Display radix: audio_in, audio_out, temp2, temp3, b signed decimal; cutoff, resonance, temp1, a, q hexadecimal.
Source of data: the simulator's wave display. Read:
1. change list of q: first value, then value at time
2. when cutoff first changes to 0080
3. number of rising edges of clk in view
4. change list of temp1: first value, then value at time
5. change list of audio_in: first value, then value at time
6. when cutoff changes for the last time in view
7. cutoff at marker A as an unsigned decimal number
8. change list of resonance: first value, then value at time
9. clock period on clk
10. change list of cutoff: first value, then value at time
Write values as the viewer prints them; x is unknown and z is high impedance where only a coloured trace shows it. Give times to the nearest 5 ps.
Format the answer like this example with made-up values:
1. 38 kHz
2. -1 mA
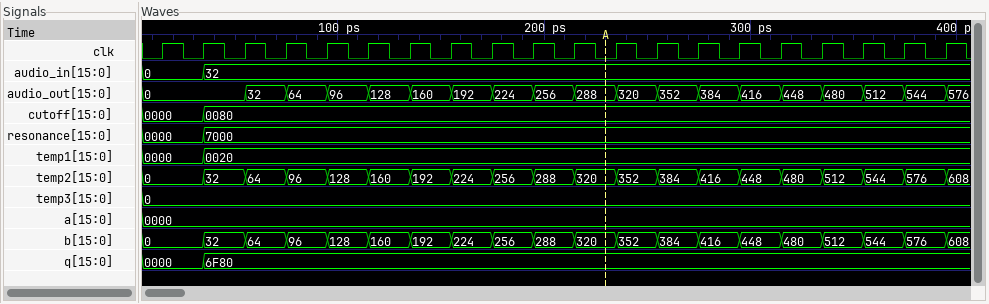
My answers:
1. 0000, 6F80 at 35 ps
2. 35 ps
3. 20
4. 0000, 0020 at 35 ps
5. 0, 32 at 35 ps
6. 35 ps
7. 128
8. 0000, 7000 at 35 ps
9. 20 ps
10. 0000, 0080 at 35 ps
